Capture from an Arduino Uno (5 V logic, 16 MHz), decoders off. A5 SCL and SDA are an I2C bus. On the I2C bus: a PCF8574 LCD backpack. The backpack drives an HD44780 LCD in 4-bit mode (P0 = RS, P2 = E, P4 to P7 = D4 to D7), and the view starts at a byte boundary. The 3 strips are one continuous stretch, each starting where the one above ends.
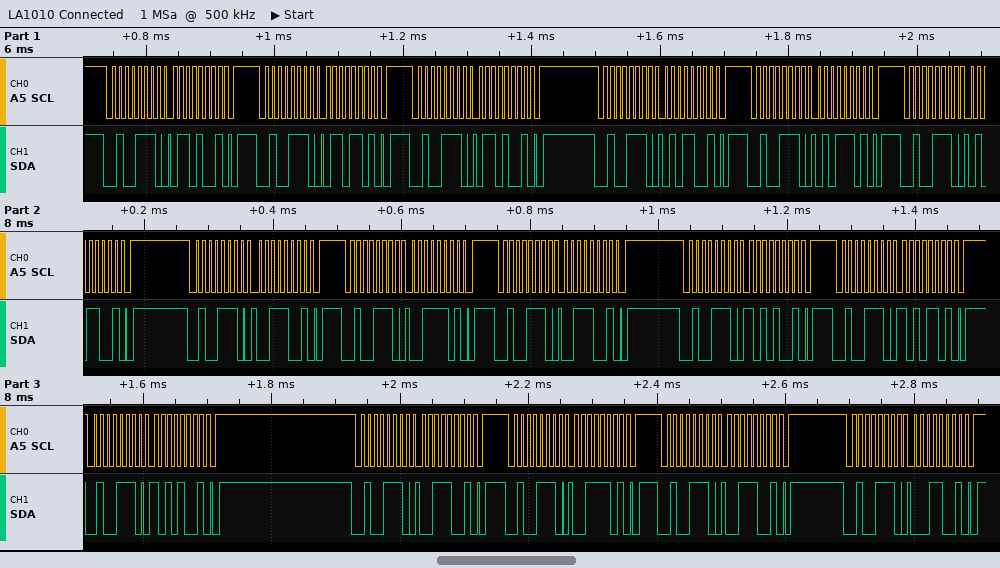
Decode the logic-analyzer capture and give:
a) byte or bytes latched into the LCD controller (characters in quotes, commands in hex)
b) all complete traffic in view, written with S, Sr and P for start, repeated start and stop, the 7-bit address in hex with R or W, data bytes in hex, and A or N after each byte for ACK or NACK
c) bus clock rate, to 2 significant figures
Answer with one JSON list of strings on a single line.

["'e' ':'", "S 27W A 69 A P S 27W A 6D A P S 27W A 69 A P S 27W A 59 A P S 27W A 5D A P S 27W A 59 A P S 27W A 39 A P S 27W A 3D A P S 27W A 39 A P S 27W A A9 A P S 27W A AD A P S 27W A A9 A P S 27W A 39 A P S 27W A 3D A P S 27W A 39 A P S 27W A 19 A P", "100 kHz"]
